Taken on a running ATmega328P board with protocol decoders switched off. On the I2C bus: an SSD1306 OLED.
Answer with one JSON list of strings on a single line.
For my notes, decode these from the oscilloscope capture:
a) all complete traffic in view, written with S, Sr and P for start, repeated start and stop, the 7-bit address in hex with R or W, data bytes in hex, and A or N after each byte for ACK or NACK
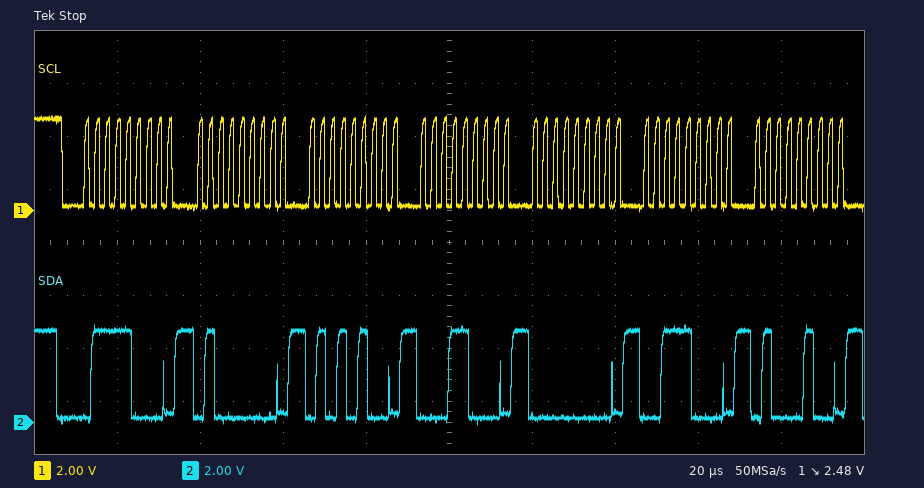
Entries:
["S 3CW A 40 A 54 A 18 A 00 A 38 A 44 A"]
